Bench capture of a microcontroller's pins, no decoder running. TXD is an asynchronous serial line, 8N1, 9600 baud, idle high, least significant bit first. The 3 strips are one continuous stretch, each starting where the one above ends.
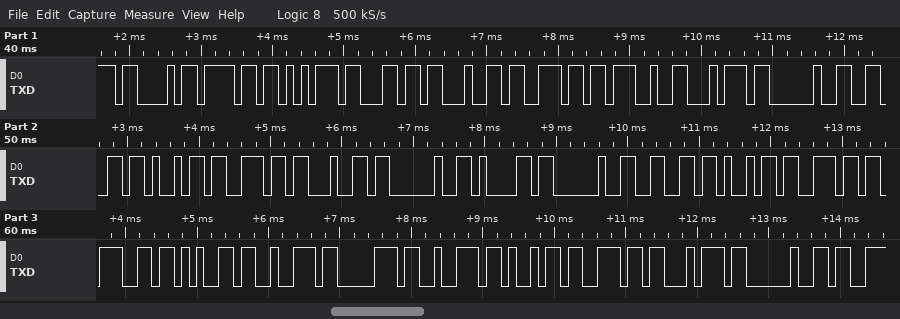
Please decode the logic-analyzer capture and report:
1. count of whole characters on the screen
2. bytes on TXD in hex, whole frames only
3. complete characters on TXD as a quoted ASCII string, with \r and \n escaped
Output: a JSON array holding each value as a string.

["28", "43 6F 75 6C 64 6E 27 74 20 66 69 6E 64 20 61 20 66 69 6E 67 65 72 70 72 69 6E 74 20", "\"Couldn't find a fingerprint \""]
